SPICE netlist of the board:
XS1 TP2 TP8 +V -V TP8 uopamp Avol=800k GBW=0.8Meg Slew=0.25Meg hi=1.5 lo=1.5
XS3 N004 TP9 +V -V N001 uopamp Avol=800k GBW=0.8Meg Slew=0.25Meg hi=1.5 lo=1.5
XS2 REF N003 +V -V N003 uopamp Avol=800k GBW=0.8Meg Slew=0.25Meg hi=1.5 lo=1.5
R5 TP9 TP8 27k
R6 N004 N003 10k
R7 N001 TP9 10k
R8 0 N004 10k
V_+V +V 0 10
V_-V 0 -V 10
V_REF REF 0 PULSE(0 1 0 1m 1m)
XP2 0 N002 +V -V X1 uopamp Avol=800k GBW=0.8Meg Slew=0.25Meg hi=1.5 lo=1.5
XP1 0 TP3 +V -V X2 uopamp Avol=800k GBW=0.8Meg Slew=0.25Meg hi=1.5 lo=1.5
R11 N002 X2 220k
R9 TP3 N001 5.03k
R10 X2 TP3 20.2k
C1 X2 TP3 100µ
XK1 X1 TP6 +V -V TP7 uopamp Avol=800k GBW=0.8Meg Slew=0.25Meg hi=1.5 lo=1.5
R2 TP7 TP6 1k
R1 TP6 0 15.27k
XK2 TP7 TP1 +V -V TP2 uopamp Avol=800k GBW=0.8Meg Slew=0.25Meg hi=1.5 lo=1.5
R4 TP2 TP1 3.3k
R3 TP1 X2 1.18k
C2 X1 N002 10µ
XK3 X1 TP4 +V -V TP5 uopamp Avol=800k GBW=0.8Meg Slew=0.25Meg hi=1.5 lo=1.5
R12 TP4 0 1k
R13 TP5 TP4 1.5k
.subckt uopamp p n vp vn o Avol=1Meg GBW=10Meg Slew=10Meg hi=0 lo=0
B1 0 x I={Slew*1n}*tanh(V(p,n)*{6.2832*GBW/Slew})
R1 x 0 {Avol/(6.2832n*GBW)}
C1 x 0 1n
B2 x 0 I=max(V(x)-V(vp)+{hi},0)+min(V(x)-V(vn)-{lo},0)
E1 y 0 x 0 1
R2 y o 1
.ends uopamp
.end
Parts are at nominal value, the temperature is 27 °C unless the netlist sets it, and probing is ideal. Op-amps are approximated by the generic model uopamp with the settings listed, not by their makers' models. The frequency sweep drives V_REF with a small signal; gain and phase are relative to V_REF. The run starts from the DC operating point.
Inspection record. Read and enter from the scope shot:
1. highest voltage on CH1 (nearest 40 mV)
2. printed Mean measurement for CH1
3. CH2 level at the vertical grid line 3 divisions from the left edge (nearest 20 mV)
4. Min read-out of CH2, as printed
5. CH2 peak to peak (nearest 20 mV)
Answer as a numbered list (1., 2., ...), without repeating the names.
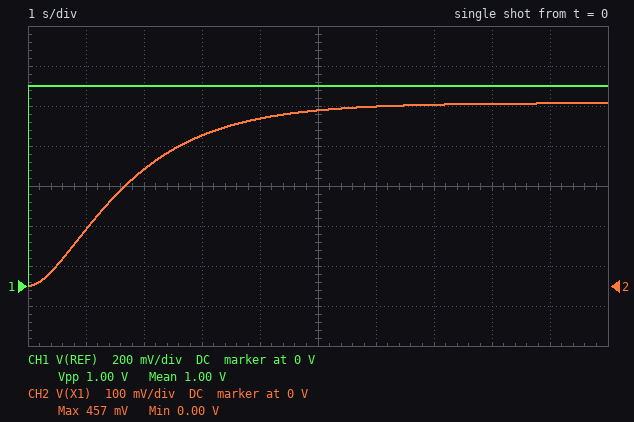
1. 1.00 V
2. 1.00 V
3. 380 mV
4. 0.00 V
5. 460 mV
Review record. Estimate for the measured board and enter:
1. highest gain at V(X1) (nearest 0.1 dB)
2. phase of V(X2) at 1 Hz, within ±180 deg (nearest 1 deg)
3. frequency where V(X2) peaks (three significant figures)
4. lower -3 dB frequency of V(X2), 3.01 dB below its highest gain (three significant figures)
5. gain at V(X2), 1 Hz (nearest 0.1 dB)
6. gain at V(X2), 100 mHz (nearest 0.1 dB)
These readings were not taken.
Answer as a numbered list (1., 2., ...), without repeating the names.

1. -6.8 dB
2. 113 deg
3. 185 mHz
4. 71.7 mHz
5. -13.7 dB
6. -6.8 dB
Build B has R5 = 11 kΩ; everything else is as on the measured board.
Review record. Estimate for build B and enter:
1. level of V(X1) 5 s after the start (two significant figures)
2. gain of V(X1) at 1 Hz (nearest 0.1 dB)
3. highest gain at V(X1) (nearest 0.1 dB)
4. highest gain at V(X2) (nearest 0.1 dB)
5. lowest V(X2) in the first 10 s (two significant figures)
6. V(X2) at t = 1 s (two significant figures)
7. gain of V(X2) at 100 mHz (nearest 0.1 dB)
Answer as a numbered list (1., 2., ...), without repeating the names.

1. 250 mV
2. -35.3 dB
3. -11.7 dB
4. -9.3 dB
5. -280 mV
6. -230 mV
7. -11.6 dB
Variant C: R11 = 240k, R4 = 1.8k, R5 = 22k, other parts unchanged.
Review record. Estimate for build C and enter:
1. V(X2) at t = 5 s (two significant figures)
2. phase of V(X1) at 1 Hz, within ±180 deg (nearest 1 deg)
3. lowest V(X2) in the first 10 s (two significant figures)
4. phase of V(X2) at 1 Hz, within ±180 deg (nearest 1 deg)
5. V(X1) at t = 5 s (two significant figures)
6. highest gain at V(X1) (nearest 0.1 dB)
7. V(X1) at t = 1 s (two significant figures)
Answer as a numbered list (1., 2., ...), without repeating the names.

1. -35 mV
2. -163 deg
3. -550 mV
4. 107 deg
5. 580 mV
6. -4.5 dB
7. 160 mV
